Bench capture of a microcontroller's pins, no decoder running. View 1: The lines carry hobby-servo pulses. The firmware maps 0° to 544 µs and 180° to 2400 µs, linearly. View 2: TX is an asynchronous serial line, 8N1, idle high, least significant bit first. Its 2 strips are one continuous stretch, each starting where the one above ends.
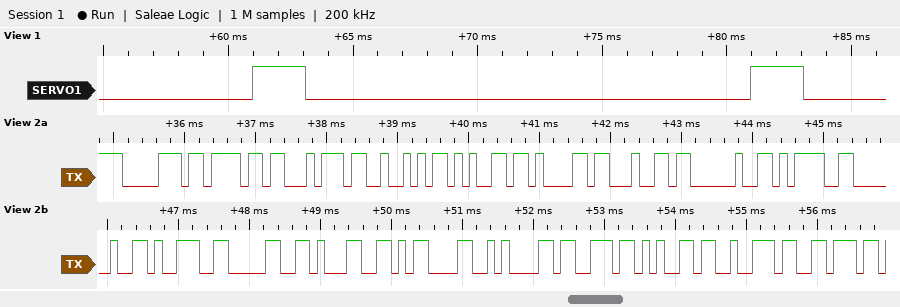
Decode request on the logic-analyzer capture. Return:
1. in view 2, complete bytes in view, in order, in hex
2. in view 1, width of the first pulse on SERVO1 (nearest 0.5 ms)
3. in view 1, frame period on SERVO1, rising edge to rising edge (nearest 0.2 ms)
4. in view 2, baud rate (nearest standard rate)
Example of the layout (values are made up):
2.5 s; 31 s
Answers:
0x70 0x6F 0x74 0x52 0x65 0x61 0x64 0x20 0x3D 0x20 0x39 0x30 0x31 0x0D 0x0A 0x73 0x65 0x72 0x76; 2.0 ms; 20.0 ms; 9600 baud
